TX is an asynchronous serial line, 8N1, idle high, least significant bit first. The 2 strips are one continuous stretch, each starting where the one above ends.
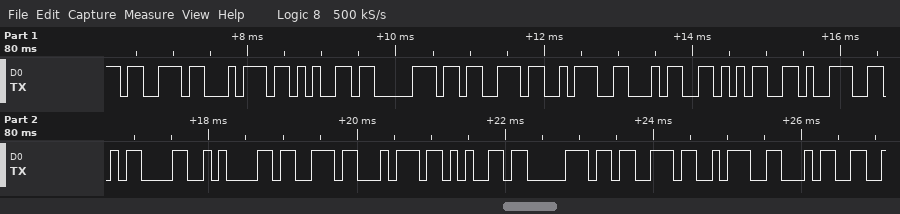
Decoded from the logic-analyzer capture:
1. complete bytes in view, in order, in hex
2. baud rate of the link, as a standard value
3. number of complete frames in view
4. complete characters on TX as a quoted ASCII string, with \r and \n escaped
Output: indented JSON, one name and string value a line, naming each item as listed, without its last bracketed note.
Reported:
{
  "complete bytes in view, in order, in hex": "73 74 65 70 73 3A 34 35 39 0D 0A 73 74 65 70 73 3A 34",
  "baud rate of the link, as a standard value": "9600 baud",
  "number of complete frames in view": "18",
  "complete characters on TX as a quoted ASCII string, with \\r and \\n escaped": "\"steps:459\\r\\nsteps:4\""
}
